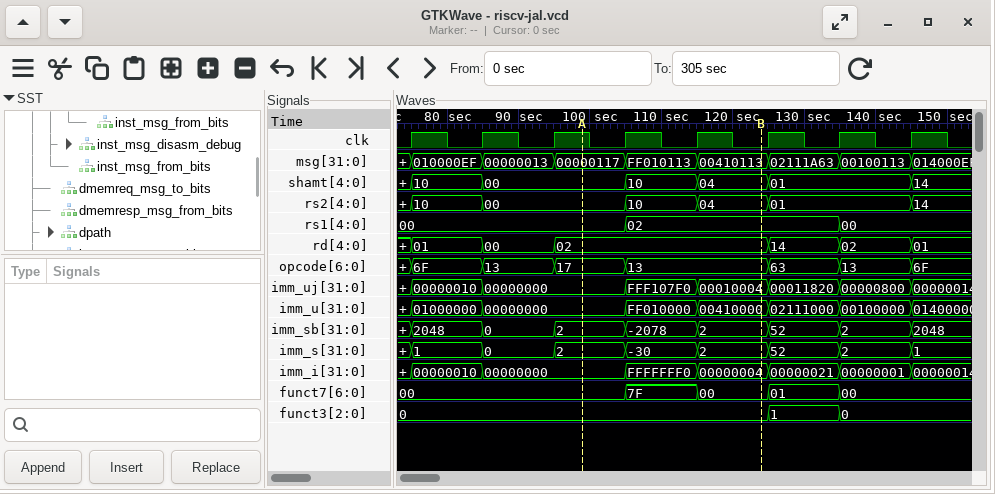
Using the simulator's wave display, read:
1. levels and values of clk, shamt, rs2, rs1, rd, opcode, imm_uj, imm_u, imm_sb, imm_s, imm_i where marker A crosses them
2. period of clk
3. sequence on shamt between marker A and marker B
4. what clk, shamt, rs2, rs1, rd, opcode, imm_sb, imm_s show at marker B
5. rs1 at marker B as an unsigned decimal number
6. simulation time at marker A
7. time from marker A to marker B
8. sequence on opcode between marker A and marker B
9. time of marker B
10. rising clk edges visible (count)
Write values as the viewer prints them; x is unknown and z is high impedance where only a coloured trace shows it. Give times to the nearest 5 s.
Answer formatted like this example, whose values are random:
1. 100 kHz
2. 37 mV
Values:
1. clk=1, shamt=00, rs2=00, rs1=00, rd=02, opcode=17, imm_uj=00000000, imm_u=00000000, imm_sb=2, imm_s=2, imm_i=00000000
2. 10 s
3. 00, 10, 04
4. clk=0, shamt=04, rs2=04, rs1=02, rd=02, opcode=13, imm_sb=2, imm_s=2
5. 2
6. 100 s
7. 25 s
8. 17, 13
9. 125 s
10. 8
